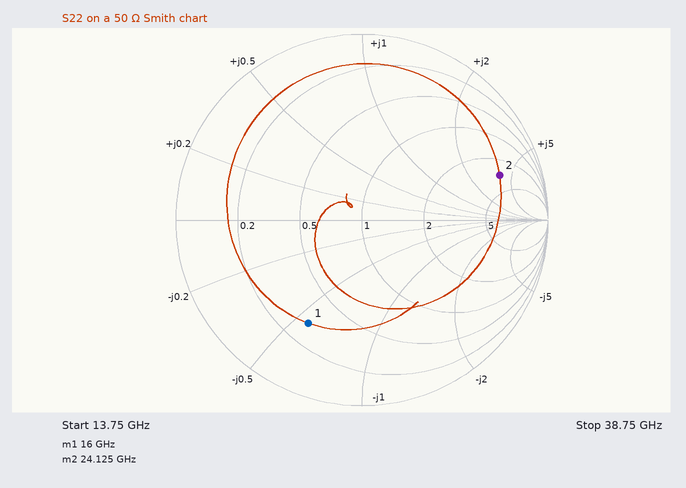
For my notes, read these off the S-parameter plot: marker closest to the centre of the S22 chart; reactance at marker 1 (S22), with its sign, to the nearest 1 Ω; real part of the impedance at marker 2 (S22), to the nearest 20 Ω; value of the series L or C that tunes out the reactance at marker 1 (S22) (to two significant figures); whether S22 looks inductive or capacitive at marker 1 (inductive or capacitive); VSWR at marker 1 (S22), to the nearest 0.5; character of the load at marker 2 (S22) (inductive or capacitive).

marker 1
-28 Ω
160 Ω
280 pH
capacitive
4.5
inductive
